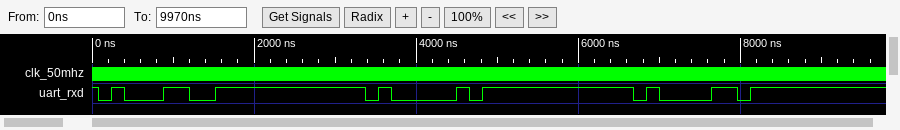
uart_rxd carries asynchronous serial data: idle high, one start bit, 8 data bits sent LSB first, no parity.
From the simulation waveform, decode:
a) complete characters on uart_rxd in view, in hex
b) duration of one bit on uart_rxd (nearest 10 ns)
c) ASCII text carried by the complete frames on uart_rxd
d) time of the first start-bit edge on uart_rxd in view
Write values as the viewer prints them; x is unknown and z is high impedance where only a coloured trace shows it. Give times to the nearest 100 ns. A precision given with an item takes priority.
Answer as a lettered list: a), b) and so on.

a) 31, 41, 61
b) 160 ns
c) "1Aa"
d) 100 ns
